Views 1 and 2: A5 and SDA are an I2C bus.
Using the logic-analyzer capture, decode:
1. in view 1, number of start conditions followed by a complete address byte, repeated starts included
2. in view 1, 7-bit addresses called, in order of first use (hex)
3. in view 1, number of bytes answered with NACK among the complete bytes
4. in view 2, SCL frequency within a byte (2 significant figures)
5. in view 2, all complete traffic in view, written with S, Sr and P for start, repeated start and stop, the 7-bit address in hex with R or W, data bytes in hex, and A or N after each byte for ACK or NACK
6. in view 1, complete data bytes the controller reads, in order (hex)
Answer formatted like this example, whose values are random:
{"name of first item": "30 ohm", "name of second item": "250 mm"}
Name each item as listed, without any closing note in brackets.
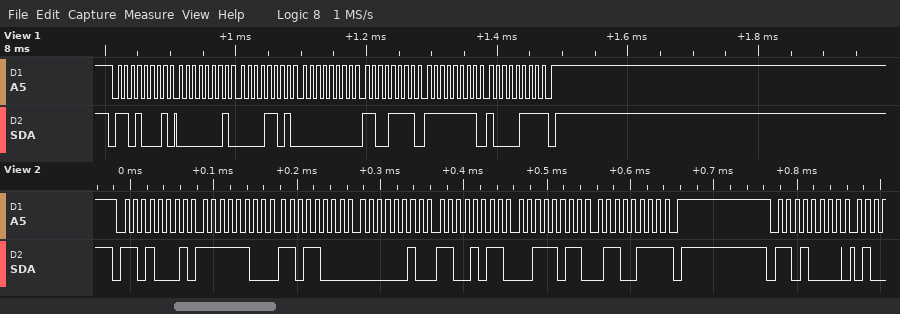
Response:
{"in view 1, number of start conditions followed by a complete address byte, repeated starts included": "1", "in view 1, 7-bit addresses called, in order of first use": "0x68", "in view 1, number of bytes answered with NACK among the complete bytes": "1", "in view 2, SCL frequency within a byte": "100 kHz", "in view 2, all complete traffic in view, written with S, Sr and P for start, repeated start and stop, the 7-bit address in hex with R or W, data bytes in hex, and A or N after each byte for ACK or NACK": "S 68R A FC A D8 A 02 A CB A 3B A 67 N P S 68W A", "in view 1, complete data bytes the controller reads, in order": "01 0D 00 CF FF 87"}
